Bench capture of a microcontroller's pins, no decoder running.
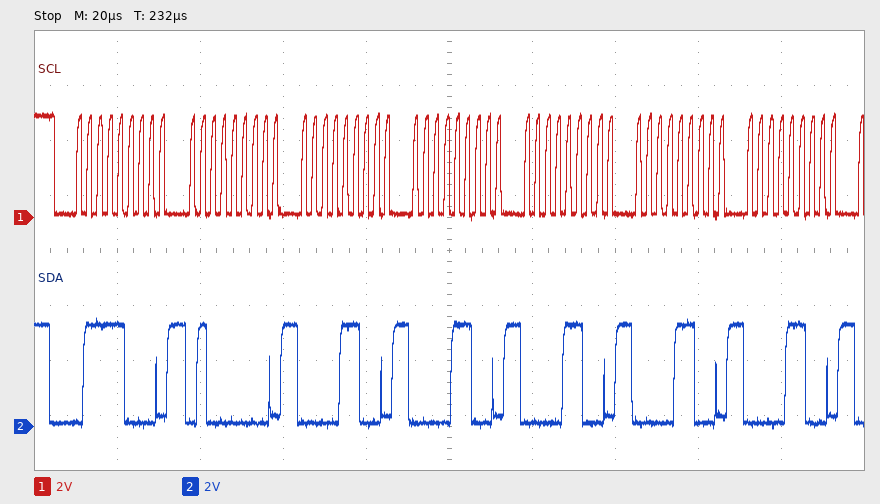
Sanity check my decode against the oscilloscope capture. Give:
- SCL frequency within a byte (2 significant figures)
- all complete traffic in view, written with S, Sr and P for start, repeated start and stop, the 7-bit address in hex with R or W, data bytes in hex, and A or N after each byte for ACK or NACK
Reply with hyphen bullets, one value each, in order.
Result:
- 400 kHz
- S 3CW A 40 A 0C A 0C A 0C A 0C A 0C A
